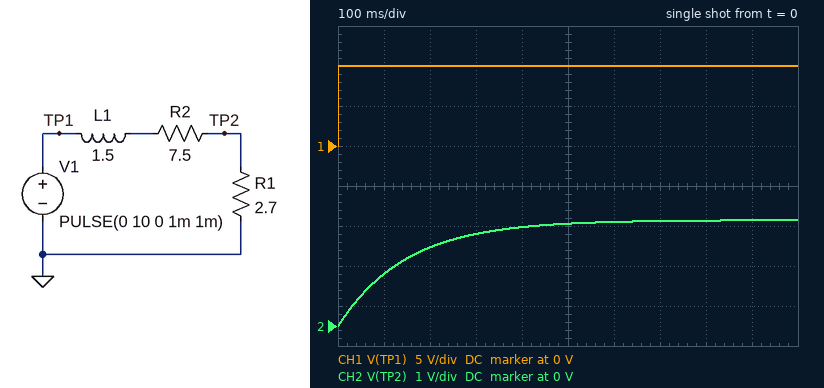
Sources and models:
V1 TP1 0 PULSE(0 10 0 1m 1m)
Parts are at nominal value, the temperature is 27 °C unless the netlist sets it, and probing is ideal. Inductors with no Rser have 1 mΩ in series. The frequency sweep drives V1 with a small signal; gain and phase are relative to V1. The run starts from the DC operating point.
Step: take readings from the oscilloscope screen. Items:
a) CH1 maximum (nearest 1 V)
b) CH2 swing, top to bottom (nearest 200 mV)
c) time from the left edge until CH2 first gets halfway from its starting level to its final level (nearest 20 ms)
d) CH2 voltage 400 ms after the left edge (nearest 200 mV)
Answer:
10 V
2.6 V
100 ms
2.4 V
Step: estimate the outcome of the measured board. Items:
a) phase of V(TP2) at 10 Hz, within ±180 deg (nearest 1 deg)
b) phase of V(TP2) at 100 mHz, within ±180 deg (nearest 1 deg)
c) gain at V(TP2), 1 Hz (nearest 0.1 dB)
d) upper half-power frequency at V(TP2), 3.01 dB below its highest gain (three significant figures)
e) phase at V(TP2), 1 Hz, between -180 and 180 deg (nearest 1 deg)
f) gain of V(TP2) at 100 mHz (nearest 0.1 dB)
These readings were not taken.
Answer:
-84 deg
-5 deg
-14.2 dB
1.08 Hz
-43 deg
-11.6 dB
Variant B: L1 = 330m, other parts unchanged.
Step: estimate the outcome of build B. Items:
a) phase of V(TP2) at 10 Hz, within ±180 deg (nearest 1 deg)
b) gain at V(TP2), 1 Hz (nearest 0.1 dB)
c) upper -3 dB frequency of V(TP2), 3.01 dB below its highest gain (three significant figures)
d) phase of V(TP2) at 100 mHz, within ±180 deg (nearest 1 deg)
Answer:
-64 deg
-11.7 dB
4.92 Hz
-1 deg
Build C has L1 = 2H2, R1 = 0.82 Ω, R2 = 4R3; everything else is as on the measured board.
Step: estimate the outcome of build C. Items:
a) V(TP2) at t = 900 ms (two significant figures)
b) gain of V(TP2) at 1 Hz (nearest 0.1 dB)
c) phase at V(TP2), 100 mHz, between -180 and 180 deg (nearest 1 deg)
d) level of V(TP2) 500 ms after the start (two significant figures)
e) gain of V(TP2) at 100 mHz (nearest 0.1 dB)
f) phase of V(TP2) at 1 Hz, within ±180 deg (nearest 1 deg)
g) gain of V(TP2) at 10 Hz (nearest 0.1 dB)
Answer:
1.4 V
-25.1 dB
-15 deg
1.1 V
-16.2 dB
-70 deg
-44.5 dB
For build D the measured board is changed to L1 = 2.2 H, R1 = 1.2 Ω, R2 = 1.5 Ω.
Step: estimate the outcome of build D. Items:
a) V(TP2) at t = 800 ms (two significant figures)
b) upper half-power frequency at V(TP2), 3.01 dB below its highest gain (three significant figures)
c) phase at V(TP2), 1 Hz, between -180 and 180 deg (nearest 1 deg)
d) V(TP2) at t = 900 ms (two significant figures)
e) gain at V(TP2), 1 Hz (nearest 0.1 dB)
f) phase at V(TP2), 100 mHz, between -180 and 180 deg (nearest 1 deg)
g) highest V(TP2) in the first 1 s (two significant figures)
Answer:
2.8 V
195 mHz
-79 deg
3.0 V
-21.4 dB
-27 deg
3.1 V
